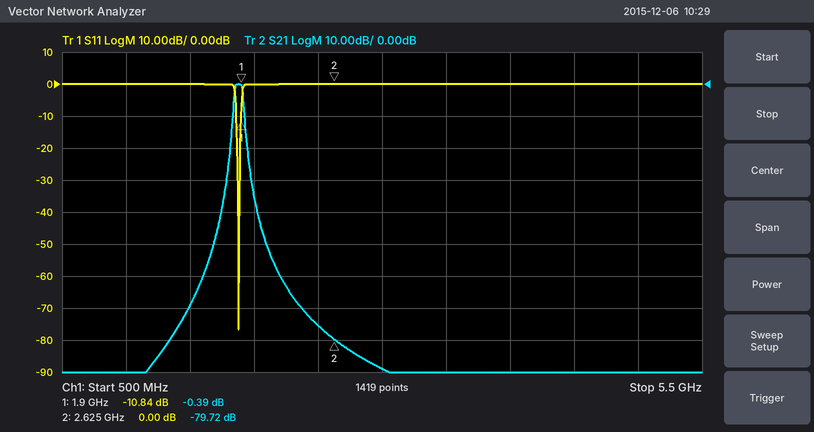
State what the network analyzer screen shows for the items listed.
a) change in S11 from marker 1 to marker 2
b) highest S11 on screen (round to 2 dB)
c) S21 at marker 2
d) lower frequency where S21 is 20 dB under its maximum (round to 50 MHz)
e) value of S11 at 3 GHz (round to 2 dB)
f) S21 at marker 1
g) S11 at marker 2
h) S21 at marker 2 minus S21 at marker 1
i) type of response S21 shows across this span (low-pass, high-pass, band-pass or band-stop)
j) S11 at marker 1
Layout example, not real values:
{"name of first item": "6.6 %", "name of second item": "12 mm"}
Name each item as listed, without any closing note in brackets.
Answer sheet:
{"change in S11 from marker 1 to marker 2": "10.84 dB", "highest S11 on screen": "0 dB", "S21 at marker 2": "-79.72 dB", "lower frequency where S21 is 20 dB under its maximum": "1.80 GHz", "value of S11 at 3 GHz": "0 dB", "S21 at marker 1": "-0.39 dB", "S11 at marker 2": "0.00 dB", "S21 at marker 2 minus S21 at marker 1": "-79.33 dB", "type of response S21 shows across this span": "band-pass", "S11 at marker 1": "-10.84 dB"}
